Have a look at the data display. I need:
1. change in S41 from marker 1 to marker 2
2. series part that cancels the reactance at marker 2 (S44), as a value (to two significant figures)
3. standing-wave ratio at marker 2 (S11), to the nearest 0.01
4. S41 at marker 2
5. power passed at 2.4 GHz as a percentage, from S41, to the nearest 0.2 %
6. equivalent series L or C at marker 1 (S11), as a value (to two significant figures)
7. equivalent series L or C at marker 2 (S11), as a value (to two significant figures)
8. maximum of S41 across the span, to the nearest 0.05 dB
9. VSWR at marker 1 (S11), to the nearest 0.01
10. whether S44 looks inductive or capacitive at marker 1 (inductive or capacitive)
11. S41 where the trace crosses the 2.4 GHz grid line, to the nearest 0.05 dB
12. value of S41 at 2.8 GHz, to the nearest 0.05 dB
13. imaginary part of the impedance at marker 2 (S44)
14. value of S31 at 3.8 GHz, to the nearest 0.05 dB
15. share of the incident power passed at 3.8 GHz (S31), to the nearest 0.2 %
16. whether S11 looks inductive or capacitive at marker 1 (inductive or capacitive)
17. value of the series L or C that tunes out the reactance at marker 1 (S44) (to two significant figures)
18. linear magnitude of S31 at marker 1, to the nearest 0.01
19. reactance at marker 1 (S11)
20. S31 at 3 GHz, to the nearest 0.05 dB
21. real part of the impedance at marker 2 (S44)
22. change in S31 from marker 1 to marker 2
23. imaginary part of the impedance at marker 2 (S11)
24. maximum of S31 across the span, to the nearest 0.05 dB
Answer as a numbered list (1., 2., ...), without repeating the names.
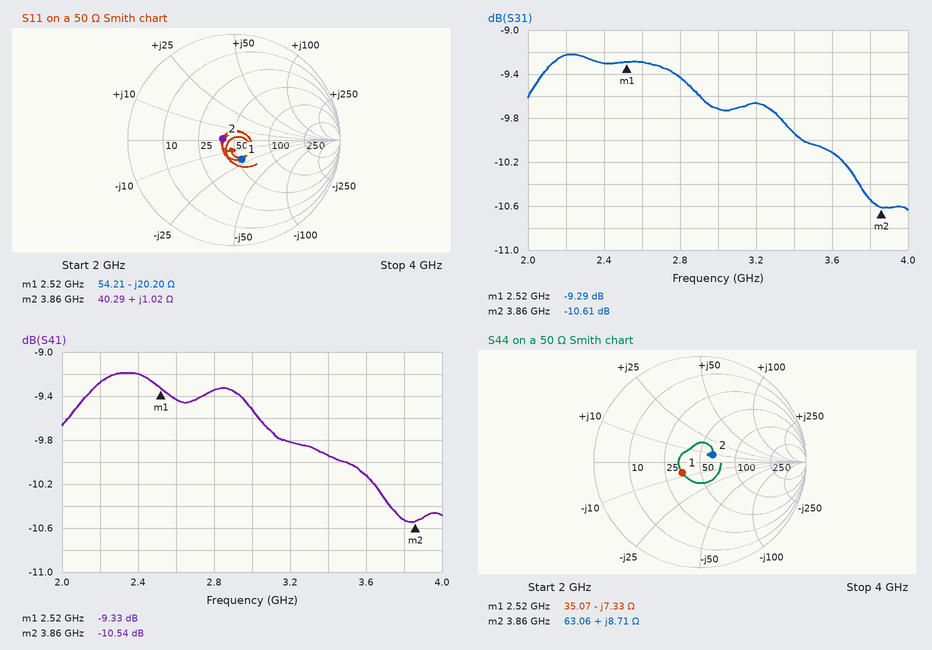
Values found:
1. -1.21 dB
2. 4.7 pF
3. 1.24
4. -10.54 dB
5. 12.0 %
6. 3.1 pF
7. 42 pH
8. -9.20 dB
9. 1.48
10. capacitive
11. -9.20 dB
12. -9.35 dB
13. +8.71 Ω
14. -10.55 dB
15. 8.8 %
16. capacitive
17. 460 pH
18. 0.34
19. -20.20 Ω
20. -9.70 dB
21. 63.06 Ω
22. -1.32 dB
23. +1.02 Ω
24. -9.20 dB
